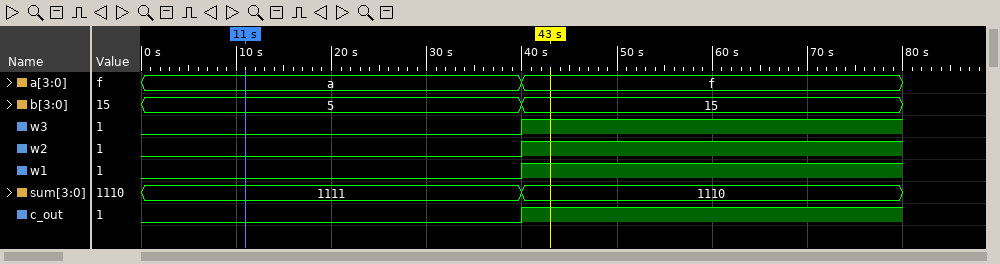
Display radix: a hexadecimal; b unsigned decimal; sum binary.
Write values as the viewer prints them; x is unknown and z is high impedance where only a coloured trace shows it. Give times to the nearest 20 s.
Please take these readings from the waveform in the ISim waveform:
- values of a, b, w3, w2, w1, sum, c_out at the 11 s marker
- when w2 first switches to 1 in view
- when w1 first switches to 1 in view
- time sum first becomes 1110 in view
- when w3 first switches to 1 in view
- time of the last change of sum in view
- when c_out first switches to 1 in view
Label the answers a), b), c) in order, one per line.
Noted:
a) a=a, b=5, w3=0, w2=0, w1=0, sum=1111, c_out=0
b) 40 s
c) 40 s
d) 40 s
e) 40 s
f) 40 s
g) 40 s
